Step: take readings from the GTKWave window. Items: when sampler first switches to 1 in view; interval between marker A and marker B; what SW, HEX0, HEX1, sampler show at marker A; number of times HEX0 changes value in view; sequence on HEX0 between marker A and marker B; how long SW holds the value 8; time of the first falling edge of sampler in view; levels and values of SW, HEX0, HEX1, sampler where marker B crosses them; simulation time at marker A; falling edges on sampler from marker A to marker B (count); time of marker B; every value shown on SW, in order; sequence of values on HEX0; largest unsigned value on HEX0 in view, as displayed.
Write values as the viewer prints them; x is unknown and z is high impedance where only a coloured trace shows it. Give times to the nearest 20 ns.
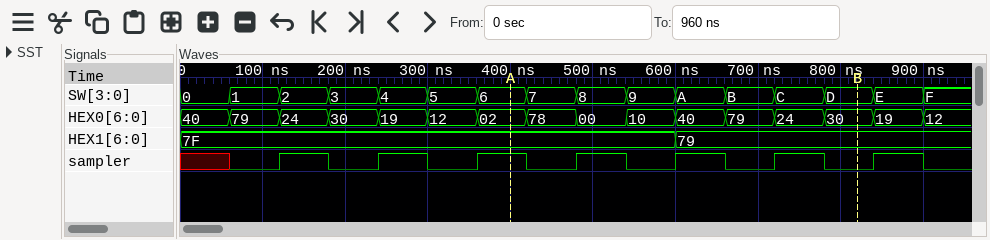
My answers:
120 ns
420 ns
SW=6, HEX0=02, HEX1=7F, sampler=1
15
02, 78, 00, 10, 40, 79, 24, 30
60 ns
180 ns
SW=D, HEX0=30, HEX1=79, sampler=0
400 ns
4
820 ns
0, 1, 2, 3, 4, 5, 6, 7, 8, 9, A, B, C, D, E, F
40, 79, 24, 30, 19, 12, 02, 78, 00, 10, 40, 79, 24, 30, 19, 12
79
